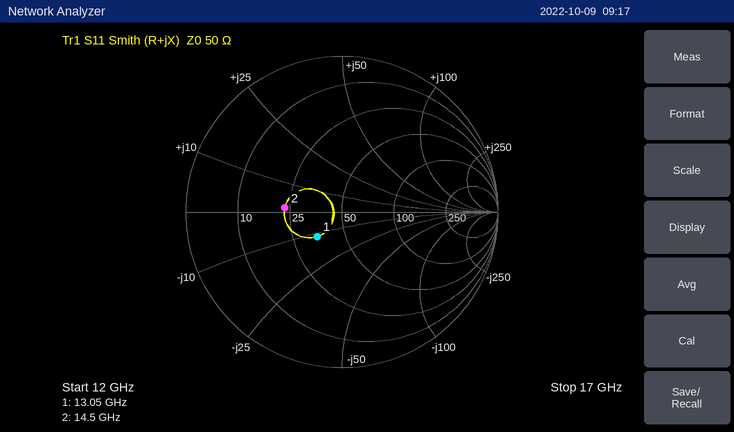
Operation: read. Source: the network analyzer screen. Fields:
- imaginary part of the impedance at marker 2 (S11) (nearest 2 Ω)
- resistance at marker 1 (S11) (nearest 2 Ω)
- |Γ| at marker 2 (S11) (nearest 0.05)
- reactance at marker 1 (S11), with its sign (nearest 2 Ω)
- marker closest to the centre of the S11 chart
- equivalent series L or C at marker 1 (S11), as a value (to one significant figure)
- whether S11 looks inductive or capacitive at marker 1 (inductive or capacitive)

+2 Ω
34 Ω
0.35
-12 Ω
marker 1
1 pF
capacitive
